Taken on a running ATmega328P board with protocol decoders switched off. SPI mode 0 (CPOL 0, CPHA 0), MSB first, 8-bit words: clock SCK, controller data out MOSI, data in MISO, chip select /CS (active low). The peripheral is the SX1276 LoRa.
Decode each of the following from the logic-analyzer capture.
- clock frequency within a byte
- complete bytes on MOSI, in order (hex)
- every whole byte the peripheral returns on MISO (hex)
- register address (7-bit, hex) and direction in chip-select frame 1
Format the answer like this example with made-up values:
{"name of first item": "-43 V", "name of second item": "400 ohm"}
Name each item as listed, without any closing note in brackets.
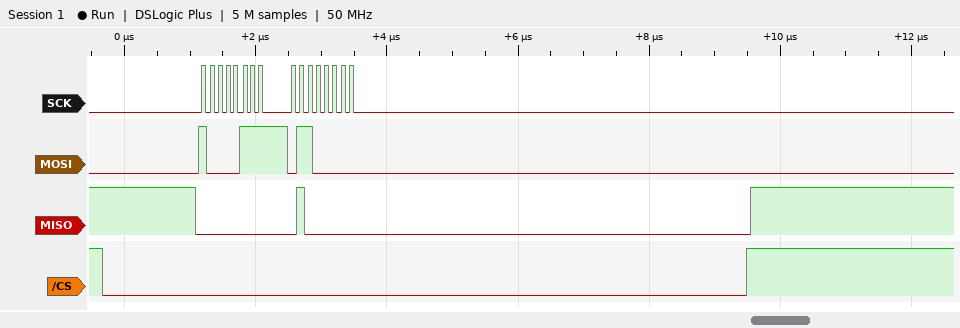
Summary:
{"clock frequency within a byte": "8 MHz", "complete bytes on MOSI, in order": "87 60", "every whole byte the peripheral returns on MISO": "00 40", "register address (7-bit, hex) and direction in chip-select frame 1": "0x07 write"}
